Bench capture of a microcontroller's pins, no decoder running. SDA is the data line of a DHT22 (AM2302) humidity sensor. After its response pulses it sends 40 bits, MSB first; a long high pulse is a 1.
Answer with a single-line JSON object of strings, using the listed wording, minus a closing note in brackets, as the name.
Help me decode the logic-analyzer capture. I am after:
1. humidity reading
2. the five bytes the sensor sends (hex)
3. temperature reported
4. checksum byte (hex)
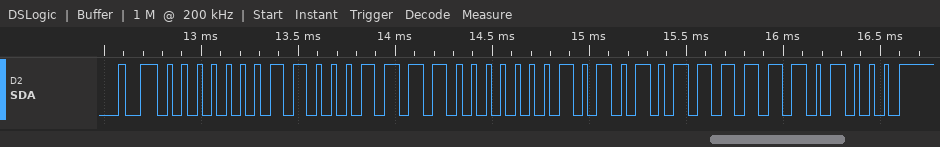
{"humidity reading": "39.9 %", "the five bytes the sensor sends": "01 8F 01 57 E8", "temperature reported": "34.3 °C", "checksum byte": "0xE8"}
